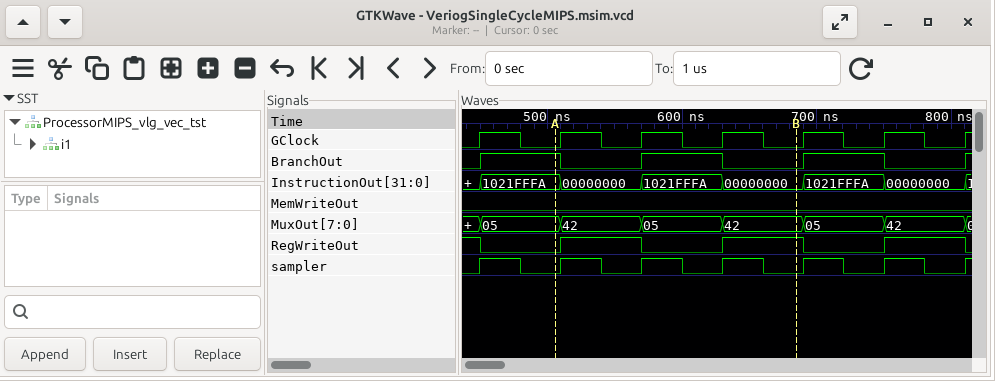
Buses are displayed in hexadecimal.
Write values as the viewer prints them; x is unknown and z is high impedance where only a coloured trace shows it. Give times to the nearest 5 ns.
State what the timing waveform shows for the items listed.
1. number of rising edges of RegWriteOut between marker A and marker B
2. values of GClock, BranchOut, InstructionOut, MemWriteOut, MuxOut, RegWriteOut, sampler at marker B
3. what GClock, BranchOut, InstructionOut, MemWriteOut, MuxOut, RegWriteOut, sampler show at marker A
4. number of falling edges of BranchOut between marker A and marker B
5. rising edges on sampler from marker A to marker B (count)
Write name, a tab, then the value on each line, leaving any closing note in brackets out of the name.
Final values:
number of rising edges of RegWriteOut between marker A and marker B	2
values of GClock, BranchOut, InstructionOut, MemWriteOut, MuxOut, RegWriteOut, sampler at marker B	GClock=0, BranchOut=0, InstructionOut=00000000, MemWriteOut=0, MuxOut=42, RegWriteOut=1, sampler=0
what GClock, BranchOut, InstructionOut, MemWriteOut, MuxOut, RegWriteOut, sampler show at marker A	GClock=0, BranchOut=1, InstructionOut=1021FFFA, MemWriteOut=0, MuxOut=05, RegWriteOut=0, sampler=0
number of falling edges of BranchOut between marker A and marker B	2
rising edges on sampler from marker A to marker B	3
